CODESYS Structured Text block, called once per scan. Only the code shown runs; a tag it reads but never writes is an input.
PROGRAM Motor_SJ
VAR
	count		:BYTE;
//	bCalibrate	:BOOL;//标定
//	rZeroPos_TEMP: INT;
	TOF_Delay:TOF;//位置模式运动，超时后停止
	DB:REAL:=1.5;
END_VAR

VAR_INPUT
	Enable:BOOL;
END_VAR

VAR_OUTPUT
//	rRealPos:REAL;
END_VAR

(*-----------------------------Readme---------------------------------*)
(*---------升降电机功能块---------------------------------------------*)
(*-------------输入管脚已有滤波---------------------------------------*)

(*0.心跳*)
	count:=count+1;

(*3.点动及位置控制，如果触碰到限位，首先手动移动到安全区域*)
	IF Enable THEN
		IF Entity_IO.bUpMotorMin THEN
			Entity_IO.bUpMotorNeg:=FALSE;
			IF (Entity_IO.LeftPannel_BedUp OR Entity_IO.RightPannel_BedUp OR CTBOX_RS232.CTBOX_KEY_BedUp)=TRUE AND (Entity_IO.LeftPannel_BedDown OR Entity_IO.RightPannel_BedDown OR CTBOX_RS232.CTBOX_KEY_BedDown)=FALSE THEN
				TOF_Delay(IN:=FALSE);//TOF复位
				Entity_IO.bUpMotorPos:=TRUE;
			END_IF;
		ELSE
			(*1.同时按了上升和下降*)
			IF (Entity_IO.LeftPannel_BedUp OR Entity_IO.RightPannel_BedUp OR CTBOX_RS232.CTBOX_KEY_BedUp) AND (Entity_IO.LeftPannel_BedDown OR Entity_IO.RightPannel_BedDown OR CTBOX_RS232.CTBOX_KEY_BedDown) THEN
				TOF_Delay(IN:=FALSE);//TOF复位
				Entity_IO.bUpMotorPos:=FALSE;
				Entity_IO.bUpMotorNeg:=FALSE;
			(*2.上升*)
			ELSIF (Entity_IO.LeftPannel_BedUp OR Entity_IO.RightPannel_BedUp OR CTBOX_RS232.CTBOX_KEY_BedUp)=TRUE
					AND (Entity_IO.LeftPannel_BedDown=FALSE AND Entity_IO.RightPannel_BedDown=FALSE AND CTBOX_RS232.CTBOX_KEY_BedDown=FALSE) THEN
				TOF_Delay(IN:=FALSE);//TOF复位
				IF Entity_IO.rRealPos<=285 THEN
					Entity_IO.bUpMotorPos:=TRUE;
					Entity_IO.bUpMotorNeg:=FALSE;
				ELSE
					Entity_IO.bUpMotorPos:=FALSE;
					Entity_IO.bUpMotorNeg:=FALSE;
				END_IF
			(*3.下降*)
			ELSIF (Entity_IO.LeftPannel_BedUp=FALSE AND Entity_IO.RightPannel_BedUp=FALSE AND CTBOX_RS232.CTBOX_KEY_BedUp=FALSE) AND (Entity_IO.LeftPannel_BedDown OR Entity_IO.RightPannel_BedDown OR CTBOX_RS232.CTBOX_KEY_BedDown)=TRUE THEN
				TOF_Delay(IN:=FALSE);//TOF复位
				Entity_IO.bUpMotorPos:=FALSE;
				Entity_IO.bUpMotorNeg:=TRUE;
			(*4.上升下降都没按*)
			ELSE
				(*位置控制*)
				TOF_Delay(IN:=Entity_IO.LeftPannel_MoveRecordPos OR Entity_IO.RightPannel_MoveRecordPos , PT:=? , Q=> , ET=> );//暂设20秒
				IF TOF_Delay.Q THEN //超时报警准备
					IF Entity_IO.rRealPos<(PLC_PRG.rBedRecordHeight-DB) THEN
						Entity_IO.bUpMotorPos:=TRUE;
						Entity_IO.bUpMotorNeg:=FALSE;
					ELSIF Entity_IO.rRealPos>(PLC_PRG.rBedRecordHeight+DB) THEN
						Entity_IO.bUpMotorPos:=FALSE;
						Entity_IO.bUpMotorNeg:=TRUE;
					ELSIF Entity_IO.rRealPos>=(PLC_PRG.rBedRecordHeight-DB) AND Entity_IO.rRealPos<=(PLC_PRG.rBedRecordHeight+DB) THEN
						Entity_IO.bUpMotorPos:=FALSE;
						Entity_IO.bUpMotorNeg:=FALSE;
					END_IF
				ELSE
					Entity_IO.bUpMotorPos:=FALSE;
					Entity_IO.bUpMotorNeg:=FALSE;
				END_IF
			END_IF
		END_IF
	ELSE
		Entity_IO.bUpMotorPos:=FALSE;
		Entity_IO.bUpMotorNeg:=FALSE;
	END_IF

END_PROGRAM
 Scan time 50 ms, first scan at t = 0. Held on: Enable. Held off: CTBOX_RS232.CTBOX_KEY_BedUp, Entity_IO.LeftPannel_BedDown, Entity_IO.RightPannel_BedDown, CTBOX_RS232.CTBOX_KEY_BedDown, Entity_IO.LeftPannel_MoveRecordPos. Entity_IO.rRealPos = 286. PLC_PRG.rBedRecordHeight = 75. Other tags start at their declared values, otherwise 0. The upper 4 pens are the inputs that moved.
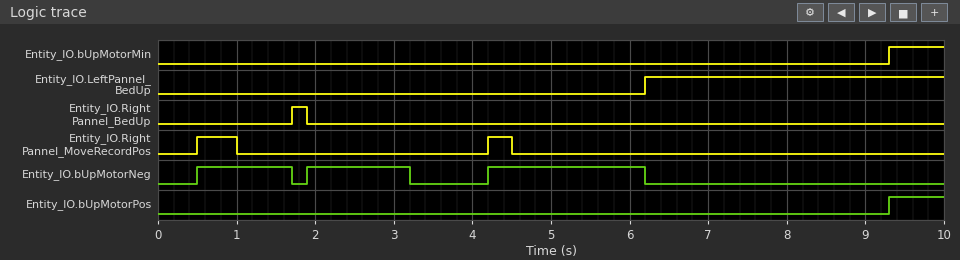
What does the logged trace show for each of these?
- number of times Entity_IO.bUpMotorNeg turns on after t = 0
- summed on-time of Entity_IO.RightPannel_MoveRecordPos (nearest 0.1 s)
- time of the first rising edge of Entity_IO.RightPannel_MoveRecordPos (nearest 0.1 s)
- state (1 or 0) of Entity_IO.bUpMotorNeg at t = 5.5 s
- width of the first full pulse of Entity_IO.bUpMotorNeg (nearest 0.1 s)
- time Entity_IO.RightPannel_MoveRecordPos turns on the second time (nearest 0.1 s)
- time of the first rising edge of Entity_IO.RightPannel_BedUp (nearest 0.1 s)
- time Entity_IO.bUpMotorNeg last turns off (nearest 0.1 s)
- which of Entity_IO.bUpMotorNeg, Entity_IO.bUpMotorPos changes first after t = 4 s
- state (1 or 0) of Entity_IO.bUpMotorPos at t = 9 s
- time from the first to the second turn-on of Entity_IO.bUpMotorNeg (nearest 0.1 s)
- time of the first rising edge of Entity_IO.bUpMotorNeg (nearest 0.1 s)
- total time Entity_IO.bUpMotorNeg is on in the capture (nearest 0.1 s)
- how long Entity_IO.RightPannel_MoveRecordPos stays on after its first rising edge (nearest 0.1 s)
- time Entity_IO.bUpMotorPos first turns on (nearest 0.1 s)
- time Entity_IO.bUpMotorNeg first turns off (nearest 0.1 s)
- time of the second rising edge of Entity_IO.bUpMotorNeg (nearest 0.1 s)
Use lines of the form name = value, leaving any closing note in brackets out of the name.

number of times Entity_IO.bUpMotorNeg turns on after t = 0 = 3
summed on-time of Entity_IO.RightPannel_MoveRecordPos = 0.8 s
time of the first rising edge of Entity_IO.RightPannel_MoveRecordPos = 0.5 s
state (1 or 0) of Entity_IO.bUpMotorNeg at t = 5.5 s = 1
width of the first full pulse of Entity_IO.bUpMotorNeg = 1.2 s
time Entity_IO.RightPannel_MoveRecordPos turns on the second time = 4.2 s
time of the first rising edge of Entity_IO.RightPannel_BedUp = 1.7 s
time Entity_IO.bUpMotorNeg last turns off = 6.2 s
which of Entity_IO.bUpMotorNeg, Entity_IO.bUpMotorPos changes first after t = 4 s = Entity_IO.bUpMotorNeg
state (1 or 0) of Entity_IO.bUpMotorPos at t = 9 s = 0
time from the first to the second turn-on of Entity_IO.bUpMotorNeg = 1.4 s
time of the first rising edge of Entity_IO.bUpMotorNeg = 0.5 s
total time Entity_IO.bUpMotorNeg is on in the capture = 4.5 s
how long Entity_IO.RightPannel_MoveRecordPos stays on after its first rising edge = 0.5 s
time Entity_IO.bUpMotorPos first turns on = 9.3 s
time Entity_IO.bUpMotorNeg first turns off = 1.7 s
time of the second rising edge of Entity_IO.bUpMotorNeg = 1.9 s
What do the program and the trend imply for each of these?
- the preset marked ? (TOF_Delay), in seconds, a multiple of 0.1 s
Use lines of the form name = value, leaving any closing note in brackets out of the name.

the preset marked ? (TOF_Delay), in seconds, a multiple of 0.1 s = 2.2 s
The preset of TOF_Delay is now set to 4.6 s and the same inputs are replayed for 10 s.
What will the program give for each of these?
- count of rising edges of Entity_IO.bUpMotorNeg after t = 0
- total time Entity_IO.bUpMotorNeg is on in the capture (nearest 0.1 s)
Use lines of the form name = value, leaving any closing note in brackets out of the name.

count of rising edges of Entity_IO.bUpMotorNeg after t = 0 = 2
total time Entity_IO.bUpMotorNeg is on in the capture = 5.5 s
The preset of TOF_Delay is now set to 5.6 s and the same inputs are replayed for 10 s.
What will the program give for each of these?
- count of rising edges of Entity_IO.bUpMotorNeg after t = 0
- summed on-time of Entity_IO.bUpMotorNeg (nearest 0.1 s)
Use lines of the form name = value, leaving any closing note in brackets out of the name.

count of rising edges of Entity_IO.bUpMotorNeg after t = 0 = 2
summed on-time of Entity_IO.bUpMotorNeg = 5.5 s
